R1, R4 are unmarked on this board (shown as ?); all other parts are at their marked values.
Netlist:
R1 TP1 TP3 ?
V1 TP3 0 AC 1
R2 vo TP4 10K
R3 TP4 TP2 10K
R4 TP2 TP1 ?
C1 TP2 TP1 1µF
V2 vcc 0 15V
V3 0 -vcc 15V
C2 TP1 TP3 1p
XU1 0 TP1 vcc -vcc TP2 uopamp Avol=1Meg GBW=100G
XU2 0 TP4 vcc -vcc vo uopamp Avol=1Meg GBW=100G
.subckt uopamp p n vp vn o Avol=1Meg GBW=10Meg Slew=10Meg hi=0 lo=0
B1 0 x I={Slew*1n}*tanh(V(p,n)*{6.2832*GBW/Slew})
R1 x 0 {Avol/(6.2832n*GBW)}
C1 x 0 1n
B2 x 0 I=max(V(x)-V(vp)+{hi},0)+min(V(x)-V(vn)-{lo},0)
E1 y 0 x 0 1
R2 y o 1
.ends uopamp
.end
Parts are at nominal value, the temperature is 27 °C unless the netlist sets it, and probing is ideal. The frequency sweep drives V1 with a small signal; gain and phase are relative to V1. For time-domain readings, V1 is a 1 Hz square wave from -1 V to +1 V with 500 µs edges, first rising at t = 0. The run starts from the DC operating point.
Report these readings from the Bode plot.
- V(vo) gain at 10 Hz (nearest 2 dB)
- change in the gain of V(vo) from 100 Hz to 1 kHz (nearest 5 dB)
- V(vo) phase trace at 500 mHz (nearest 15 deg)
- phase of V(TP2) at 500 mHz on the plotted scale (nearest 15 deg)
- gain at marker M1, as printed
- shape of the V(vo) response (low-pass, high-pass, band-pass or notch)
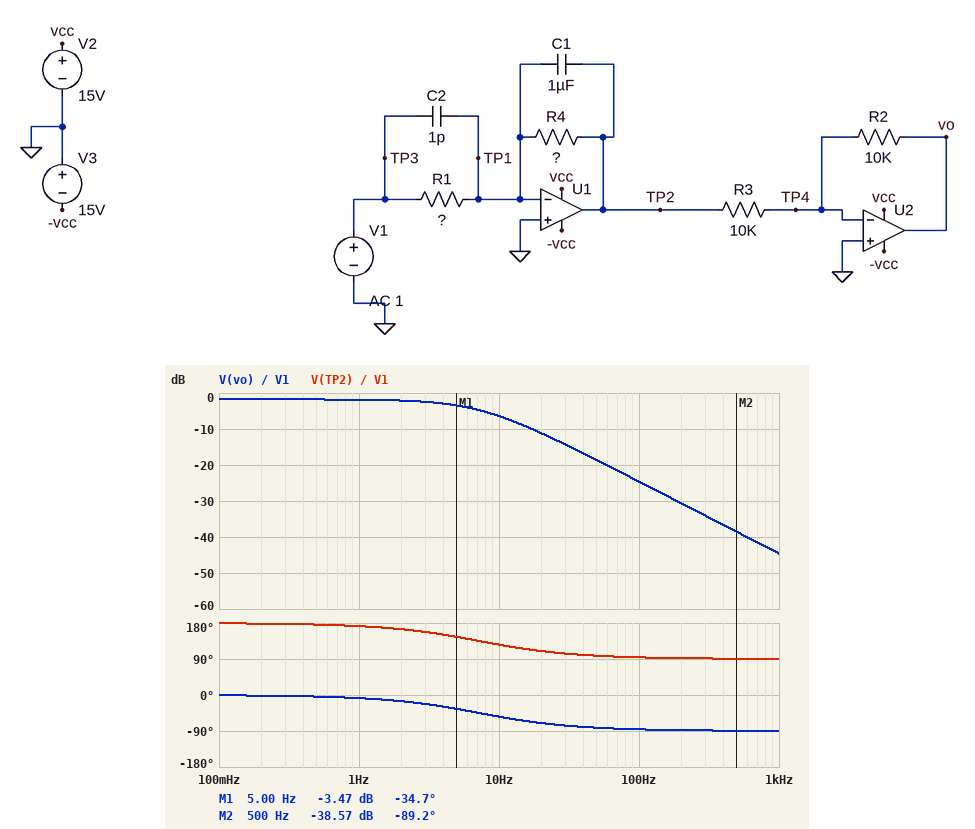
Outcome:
-6 dB
-20 dB
0 deg
180 deg
-3.47 dB
low-pass
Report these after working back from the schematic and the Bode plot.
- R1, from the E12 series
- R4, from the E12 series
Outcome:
27 kΩ
22 kΩ
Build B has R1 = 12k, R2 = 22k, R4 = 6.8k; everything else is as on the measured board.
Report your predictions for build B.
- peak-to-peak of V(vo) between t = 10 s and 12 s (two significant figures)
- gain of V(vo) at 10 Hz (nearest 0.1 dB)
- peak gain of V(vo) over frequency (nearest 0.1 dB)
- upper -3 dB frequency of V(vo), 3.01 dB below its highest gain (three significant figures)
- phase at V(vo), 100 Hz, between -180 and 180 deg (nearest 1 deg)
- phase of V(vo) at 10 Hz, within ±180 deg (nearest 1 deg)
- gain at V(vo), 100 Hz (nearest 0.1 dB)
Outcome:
2.5 V
1.2 dB
1.9 dB
23.4 Hz
-77 deg
-23 deg
-10.9 dB
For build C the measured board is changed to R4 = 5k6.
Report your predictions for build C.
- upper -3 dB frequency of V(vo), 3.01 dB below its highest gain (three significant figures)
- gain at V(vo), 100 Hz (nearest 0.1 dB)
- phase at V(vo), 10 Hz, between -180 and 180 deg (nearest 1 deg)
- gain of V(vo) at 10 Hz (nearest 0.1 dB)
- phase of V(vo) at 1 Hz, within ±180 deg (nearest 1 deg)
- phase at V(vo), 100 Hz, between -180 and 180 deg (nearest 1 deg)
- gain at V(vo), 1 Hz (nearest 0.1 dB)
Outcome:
28.4 Hz
-24.9 dB
-19 deg
-14.2 dB
-2 deg
-74 deg
-13.7 dB
